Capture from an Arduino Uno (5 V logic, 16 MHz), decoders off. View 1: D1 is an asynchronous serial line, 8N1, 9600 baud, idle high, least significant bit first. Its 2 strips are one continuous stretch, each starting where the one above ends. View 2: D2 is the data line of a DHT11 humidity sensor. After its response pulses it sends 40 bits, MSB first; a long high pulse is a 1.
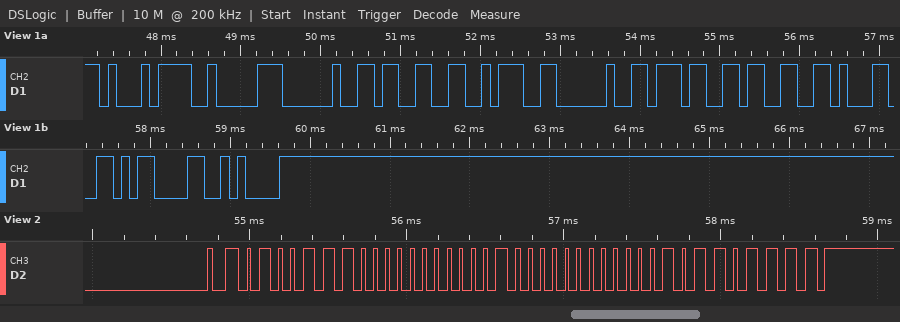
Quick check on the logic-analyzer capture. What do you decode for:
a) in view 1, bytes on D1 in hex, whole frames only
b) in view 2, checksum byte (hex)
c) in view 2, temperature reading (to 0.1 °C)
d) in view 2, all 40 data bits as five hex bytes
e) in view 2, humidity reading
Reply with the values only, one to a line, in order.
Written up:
D1 82 20 33 3A 20 37 33 31 0D 0A
0x6F
32.1 °C
4E 00 20 01 6F
78 %
